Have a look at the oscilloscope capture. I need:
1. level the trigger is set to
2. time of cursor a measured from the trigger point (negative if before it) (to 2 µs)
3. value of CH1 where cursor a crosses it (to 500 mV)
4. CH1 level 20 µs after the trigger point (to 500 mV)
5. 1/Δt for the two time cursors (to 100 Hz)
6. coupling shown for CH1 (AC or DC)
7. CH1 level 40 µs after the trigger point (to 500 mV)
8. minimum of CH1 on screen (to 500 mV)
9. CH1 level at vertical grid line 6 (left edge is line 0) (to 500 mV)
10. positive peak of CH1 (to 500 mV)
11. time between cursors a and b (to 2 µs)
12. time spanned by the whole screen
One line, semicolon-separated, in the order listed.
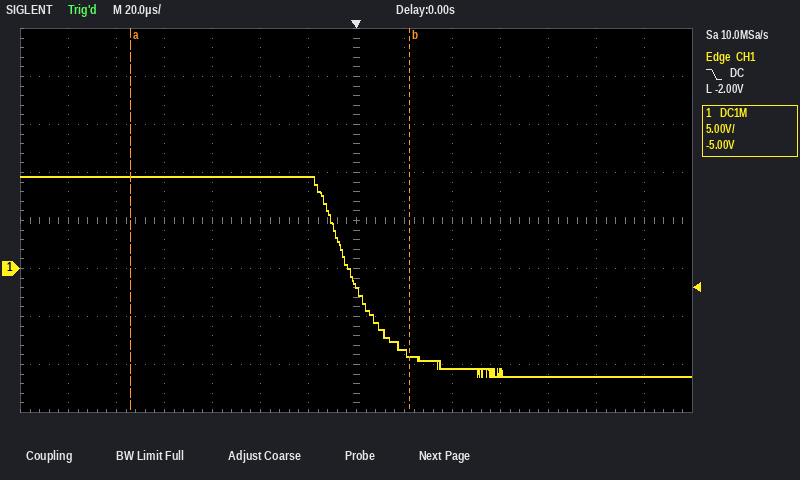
-2.00 V; -94 µs; 9.5 V; -8.5 V; 8.6 kHz; DC; -10.5 V; -11.0 V; 9.5 V; 9.5 V; 116 µs; 280 µs
